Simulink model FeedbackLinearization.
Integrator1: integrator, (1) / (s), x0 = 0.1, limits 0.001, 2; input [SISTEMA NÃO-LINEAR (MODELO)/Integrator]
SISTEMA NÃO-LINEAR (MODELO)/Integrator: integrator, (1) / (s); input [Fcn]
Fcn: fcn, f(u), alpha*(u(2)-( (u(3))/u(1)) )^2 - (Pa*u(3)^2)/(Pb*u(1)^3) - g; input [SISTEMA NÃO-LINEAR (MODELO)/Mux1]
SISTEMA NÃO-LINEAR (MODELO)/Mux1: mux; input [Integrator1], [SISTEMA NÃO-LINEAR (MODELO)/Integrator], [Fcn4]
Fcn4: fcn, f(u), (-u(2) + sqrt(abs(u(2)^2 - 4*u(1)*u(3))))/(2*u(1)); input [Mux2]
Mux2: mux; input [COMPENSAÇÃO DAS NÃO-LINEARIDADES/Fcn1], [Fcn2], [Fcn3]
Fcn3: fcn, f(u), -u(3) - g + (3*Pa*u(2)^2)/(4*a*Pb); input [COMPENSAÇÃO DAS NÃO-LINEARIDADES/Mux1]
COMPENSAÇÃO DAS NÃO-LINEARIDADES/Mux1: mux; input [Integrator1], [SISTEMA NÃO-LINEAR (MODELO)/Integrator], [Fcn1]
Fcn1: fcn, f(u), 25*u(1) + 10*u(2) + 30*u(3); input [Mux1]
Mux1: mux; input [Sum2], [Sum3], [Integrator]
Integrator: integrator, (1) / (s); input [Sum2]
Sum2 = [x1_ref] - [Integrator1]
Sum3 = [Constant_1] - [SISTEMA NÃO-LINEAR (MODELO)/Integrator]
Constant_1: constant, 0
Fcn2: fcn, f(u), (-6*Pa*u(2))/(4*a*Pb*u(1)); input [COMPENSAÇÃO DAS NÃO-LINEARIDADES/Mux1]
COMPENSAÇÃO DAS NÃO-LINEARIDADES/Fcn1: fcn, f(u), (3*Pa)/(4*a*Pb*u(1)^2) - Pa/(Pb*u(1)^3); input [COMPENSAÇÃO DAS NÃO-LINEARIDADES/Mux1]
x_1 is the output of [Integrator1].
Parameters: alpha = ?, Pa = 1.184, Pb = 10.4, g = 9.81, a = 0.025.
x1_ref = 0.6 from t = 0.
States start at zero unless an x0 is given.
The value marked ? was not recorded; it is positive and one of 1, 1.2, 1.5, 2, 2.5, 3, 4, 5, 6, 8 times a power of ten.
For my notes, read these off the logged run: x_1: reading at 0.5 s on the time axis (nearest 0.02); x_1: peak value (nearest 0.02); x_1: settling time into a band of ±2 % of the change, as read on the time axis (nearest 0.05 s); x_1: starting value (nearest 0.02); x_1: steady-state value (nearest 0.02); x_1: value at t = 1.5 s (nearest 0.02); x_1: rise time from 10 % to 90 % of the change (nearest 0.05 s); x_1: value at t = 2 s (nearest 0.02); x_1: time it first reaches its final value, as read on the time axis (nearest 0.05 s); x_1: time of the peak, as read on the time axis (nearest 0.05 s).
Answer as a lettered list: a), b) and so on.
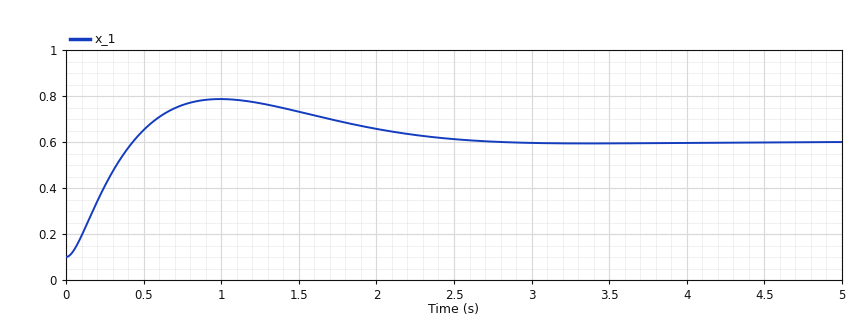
a) 0.66
b) 0.78
c) 2.55 s
d) 0.10
e) 0.60
f) 0.74
g) 0.30 s
h) 0.66
i) 0.45 s
j) 1.00 s
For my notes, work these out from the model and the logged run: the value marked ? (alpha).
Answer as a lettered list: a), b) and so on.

a) 5
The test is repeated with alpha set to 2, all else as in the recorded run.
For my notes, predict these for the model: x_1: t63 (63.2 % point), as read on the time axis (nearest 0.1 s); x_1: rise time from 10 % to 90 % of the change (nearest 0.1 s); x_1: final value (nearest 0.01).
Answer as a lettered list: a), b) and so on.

a) 0.4 s
b) 0.3 s
c) 0.00
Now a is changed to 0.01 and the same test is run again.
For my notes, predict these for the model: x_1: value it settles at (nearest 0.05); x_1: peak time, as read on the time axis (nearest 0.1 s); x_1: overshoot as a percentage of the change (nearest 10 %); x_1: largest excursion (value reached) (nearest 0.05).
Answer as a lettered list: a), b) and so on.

a) 0.60
b) 1.7 s
c) 20 %
d) 0.70
